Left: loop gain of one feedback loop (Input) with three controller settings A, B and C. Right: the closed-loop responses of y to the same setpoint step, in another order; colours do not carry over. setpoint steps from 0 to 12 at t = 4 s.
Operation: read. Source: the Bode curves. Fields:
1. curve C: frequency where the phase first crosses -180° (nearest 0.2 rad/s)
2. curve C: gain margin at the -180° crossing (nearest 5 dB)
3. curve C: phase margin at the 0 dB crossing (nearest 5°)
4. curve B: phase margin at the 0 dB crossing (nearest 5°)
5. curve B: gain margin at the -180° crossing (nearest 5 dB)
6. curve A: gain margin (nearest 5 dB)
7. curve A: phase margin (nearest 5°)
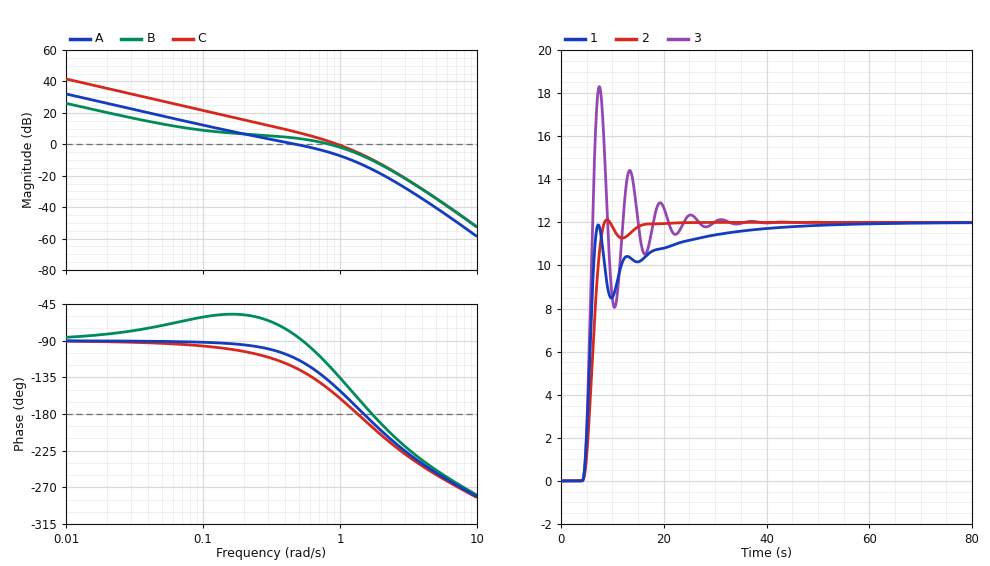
1.4 rad/s
5 dB
20°
60°
10 dB
15 dB
70°
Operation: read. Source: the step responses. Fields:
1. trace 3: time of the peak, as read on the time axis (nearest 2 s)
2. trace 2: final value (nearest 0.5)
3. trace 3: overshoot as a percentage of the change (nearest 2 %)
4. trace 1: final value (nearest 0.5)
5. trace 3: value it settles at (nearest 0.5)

8 s
12.0
52 %
12.0
12.0
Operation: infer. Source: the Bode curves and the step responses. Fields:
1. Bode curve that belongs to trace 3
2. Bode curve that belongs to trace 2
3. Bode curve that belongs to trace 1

C
A
B
